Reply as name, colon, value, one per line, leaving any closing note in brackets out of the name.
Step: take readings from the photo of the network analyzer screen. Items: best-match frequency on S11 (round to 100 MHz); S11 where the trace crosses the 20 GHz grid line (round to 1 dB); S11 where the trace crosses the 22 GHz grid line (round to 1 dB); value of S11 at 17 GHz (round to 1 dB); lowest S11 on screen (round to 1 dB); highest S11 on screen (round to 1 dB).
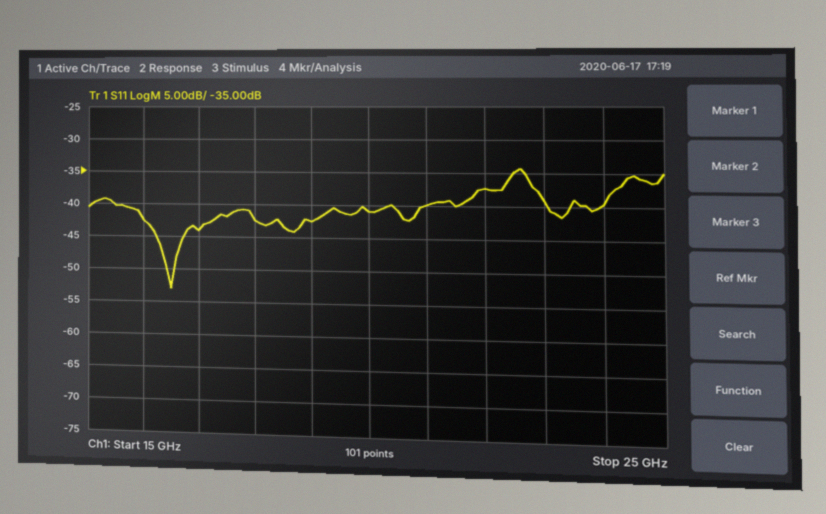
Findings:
best-match frequency on S11: 16.5 GHz
S11 where the trace crosses the 20 GHz grid line: -41 dB
S11 where the trace crosses the 22 GHz grid line: -37 dB
value of S11 at 17 GHz: -44 dB
lowest S11 on screen: -53 dB
highest S11 on screen: -34 dB
